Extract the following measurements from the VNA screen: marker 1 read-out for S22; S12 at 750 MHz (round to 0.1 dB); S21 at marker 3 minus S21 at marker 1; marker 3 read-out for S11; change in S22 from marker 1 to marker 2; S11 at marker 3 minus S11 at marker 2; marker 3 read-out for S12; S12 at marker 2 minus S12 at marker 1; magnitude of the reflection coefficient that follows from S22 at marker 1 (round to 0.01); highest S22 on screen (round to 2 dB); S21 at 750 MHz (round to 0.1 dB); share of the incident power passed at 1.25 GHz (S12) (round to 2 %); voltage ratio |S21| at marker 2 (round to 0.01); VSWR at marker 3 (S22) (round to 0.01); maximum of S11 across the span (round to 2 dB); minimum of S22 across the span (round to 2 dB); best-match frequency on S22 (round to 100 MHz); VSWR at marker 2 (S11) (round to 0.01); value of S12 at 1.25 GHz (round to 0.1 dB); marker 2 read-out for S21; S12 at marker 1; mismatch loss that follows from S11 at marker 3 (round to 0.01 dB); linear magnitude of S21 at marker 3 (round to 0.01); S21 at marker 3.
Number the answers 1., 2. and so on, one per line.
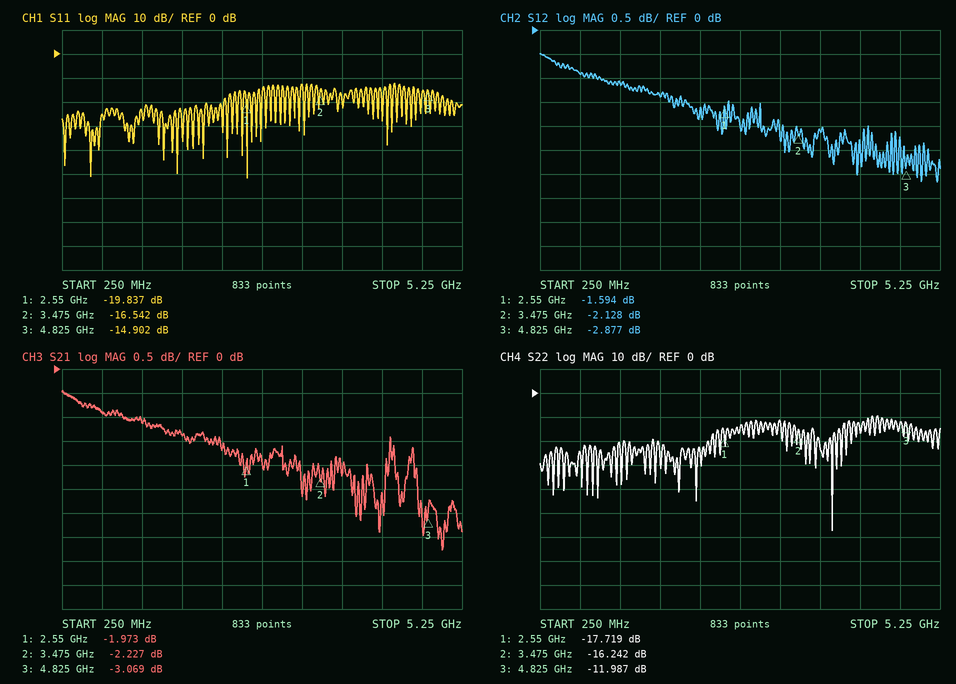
1. -17.719 dB
2. -0.9 dB
3. -1.096 dB
4. -14.902 dB
5. 1.477 dB
6. 1.640 dB
7. -2.877 dB
8. -0.534 dB
9. 0.13
10. -10 dB
11. -0.9 dB
12. 78 %
13. 0.77
14. 1.67
15. -12 dB
16. -58 dB
17. 3.9 GHz
18. 1.35
19. -1.1 dB
20. -2.227 dB
21. -1.594 dB
22. 0.14 dB
23. 0.70
24. -3.069 dB
